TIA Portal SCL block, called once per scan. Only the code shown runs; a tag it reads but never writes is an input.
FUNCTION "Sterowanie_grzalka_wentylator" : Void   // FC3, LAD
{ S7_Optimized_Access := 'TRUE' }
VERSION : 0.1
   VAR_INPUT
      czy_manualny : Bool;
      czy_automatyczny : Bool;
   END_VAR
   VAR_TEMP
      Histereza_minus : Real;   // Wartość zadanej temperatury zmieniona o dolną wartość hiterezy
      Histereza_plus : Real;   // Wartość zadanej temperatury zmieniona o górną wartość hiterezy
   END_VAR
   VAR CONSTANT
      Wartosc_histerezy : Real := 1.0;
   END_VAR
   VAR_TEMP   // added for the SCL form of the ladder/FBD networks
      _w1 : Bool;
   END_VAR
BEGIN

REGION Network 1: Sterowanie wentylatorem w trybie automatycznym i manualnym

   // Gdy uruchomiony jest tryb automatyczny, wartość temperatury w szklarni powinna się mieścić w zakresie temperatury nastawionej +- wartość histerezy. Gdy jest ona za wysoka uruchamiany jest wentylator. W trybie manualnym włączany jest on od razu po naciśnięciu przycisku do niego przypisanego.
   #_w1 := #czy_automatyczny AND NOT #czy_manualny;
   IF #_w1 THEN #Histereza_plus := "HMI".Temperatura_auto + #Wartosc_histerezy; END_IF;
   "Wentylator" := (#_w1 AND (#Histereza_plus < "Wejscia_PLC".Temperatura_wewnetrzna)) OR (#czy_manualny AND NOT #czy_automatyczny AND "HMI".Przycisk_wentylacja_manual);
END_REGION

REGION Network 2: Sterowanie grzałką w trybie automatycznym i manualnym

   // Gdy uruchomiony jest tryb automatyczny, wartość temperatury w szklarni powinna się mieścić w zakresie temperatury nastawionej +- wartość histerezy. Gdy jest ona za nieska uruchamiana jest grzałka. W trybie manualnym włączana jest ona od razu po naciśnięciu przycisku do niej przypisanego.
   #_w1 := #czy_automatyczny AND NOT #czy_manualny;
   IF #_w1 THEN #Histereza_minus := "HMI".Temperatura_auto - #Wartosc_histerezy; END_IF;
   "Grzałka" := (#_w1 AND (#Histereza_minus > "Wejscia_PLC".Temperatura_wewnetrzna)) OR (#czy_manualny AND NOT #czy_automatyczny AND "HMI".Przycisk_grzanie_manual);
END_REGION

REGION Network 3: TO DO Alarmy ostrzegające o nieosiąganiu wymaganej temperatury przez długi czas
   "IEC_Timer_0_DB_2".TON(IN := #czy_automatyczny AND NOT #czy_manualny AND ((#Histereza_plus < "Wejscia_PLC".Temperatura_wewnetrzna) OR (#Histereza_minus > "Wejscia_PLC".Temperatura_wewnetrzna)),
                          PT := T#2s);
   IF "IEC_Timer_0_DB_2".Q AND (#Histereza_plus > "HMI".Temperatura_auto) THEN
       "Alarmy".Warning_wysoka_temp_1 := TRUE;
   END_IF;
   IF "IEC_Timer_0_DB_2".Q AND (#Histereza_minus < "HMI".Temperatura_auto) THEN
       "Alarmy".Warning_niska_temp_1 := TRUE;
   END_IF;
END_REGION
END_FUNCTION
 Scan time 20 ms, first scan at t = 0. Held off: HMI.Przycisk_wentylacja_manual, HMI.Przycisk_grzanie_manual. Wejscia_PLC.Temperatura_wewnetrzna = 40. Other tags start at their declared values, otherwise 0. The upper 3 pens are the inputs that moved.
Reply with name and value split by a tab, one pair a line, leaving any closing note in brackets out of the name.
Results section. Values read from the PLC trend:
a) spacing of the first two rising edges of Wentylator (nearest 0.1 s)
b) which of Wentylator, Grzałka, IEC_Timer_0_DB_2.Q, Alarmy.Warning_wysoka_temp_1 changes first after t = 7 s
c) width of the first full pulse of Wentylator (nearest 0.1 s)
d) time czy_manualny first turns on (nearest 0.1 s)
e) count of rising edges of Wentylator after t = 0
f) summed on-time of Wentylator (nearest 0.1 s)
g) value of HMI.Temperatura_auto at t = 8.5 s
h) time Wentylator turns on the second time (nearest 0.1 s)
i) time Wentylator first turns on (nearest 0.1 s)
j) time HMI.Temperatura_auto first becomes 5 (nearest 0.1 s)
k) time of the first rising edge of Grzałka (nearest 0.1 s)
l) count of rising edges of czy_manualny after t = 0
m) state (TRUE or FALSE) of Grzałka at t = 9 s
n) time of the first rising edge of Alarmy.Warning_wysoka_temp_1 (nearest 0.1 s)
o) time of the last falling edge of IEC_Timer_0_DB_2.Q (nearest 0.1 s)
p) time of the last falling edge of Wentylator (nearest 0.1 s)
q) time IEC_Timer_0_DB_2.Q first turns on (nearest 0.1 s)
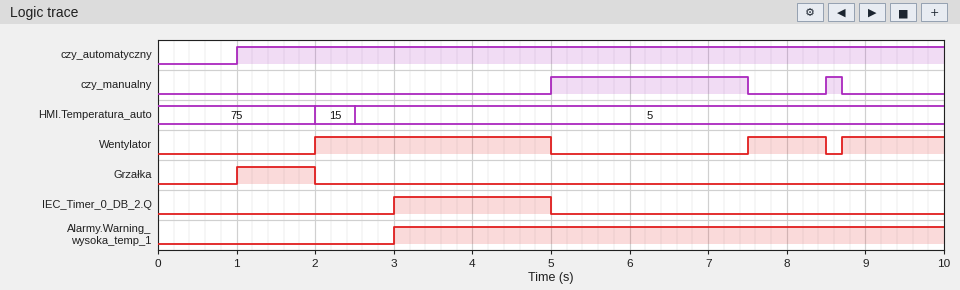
spacing of the first two rising edges of Wentylator	5.5 s
which of Wentylator, Grzałka, IEC_Timer_0_DB_2.Q, Alarmy.Warning_wysoka_temp_1 changes first after t = 7 s	Wentylator
width of the first full pulse of Wentylator	3.0 s
time czy_manualny first turns on	5.0 s
count of rising edges of Wentylator after t = 0	3
summed on-time of Wentylator	5.3 s
value of HMI.Temperatura_auto at t = 8.5 s	5
time Wentylator turns on the second time	7.5 s
time Wentylator first turns on	2.0 s
time HMI.Temperatura_auto first becomes 5	2.5 s
time of the first rising edge of Grzałka	1.0 s
count of rising edges of czy_manualny after t = 0	2
state (TRUE or FALSE) of Grzałka at t = 9 s	FALSE
time of the first rising edge of Alarmy.Warning_wysoka_temp_1	3.0 s
time of the last falling edge of IEC_Timer_0_DB_2.Q	5.0 s
time of the last falling edge of Wentylator	8.5 s
time IEC_Timer_0_DB_2.Q first turns on	3.0 s
